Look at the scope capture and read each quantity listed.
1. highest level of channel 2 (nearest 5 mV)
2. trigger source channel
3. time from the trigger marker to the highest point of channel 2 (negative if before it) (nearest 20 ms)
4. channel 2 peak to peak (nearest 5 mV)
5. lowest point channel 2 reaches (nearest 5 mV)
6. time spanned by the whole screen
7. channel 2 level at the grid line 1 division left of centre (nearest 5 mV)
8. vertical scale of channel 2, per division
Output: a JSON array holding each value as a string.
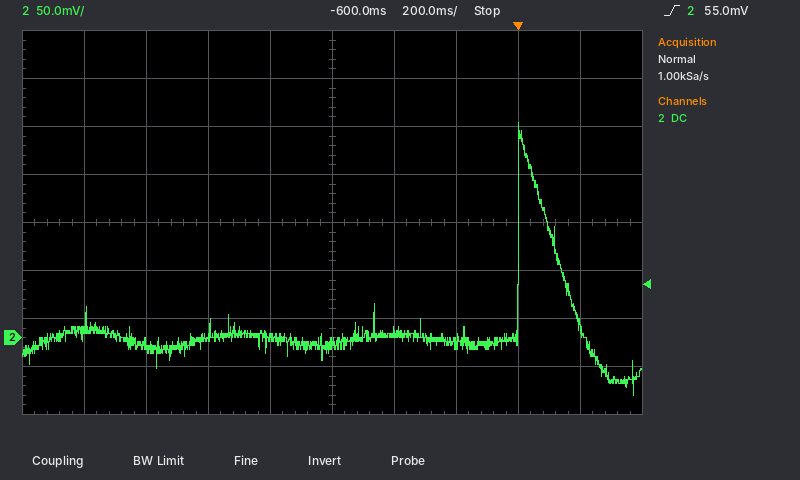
["225 mV", "channel 2", "0 ms", "285 mV", "-60 mV", "2 s", "0 mV", "50 mV"]
